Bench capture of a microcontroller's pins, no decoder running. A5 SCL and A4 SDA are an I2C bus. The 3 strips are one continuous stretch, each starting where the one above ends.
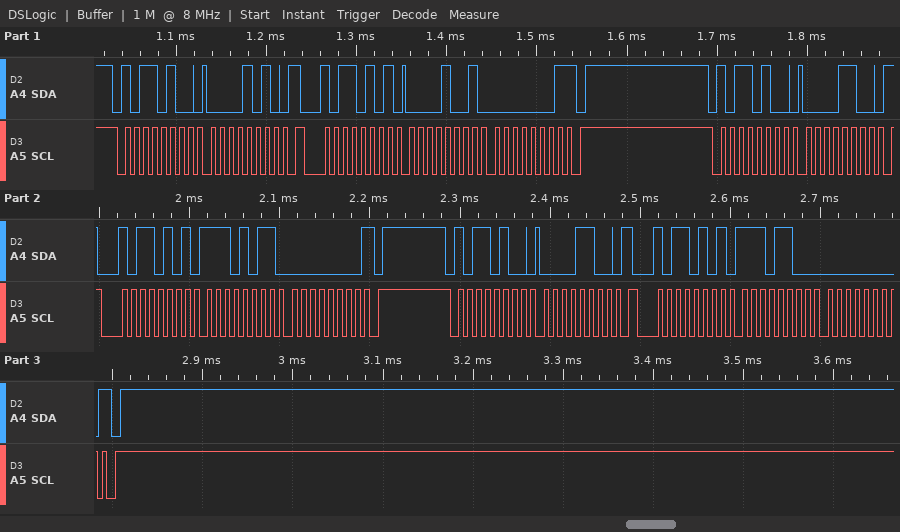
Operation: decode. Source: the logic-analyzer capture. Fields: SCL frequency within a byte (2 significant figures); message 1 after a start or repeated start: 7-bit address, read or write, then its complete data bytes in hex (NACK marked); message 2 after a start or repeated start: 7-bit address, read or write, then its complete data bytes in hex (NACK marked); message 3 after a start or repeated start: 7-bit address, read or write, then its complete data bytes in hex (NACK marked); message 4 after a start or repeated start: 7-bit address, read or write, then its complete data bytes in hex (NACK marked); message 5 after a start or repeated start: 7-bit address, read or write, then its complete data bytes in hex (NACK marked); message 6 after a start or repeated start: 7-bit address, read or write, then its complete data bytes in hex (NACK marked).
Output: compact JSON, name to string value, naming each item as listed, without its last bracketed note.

{"SCL frequency within a byte": "100 kHz", "message 1 after a start or repeated start: 7-bit address, read or write, then its complete data bytes in hex": "0x5A write: 0A", "message 2 after a start or repeated start: 7-bit address, read or write, then its complete data bytes in hex": "0x5A read: 09 01 NACK", "message 3 after a start or repeated start: 7-bit address, read or write, then its complete data bytes in hex": "0x5A write: 0C", "message 4 after a start or repeated start: 7-bit address, read or write, then its complete data bytes in hex": "0x5A read: EB 00 NACK", "message 5 after a start or repeated start: 7-bit address, read or write, then its complete data bytes in hex": "0x5A write: 0C", "message 6 after a start or repeated start: 7-bit address, read or write, then its complete data bytes in hex": "0x5A read: EC 00 NACK"}
